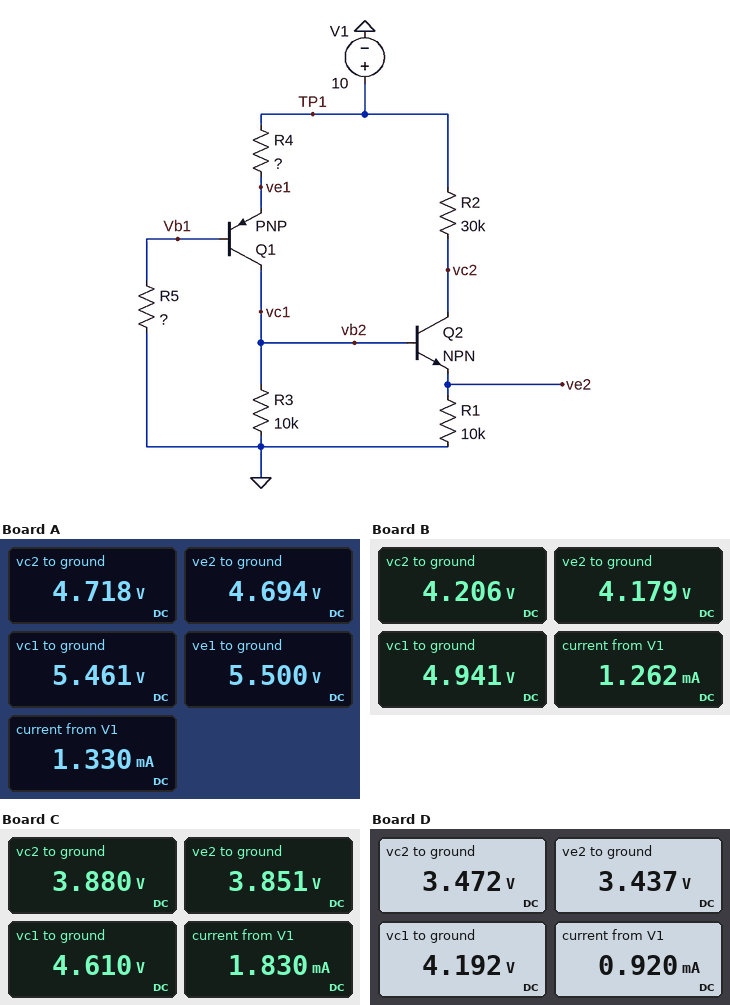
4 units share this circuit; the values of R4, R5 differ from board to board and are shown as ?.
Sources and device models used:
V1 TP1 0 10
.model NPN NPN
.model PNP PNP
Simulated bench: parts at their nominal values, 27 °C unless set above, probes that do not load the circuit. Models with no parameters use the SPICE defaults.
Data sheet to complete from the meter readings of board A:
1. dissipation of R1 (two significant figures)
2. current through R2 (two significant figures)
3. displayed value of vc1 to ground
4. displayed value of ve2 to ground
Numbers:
2.2 mW
180 µA
5.461 V
4.694 V
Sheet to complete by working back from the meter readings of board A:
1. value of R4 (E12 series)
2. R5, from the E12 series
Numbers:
3.9 kΩ
15 kΩ
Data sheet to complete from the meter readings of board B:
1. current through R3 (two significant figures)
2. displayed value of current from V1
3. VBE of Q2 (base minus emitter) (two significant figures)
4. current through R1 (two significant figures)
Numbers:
490 µA
1.262 mA
760 mV
420 µA
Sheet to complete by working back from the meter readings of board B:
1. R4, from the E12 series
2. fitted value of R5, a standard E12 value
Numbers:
4.7 kΩ
12 kΩ
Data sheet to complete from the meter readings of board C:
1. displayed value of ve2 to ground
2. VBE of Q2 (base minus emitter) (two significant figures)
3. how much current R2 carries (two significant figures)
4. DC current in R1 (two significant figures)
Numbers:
3.851 V
760 mV
200 µA
390 µA
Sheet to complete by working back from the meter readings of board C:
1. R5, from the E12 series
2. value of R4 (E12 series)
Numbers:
3.9 kΩ
3.3 kΩ
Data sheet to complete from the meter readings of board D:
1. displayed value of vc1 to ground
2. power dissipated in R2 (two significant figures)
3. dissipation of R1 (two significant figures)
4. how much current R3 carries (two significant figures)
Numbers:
4.192 V
1.4 mW
1.2 mW
420 µA
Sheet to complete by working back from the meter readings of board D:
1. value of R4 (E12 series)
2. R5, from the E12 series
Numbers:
8.2 kΩ
22 kΩ
